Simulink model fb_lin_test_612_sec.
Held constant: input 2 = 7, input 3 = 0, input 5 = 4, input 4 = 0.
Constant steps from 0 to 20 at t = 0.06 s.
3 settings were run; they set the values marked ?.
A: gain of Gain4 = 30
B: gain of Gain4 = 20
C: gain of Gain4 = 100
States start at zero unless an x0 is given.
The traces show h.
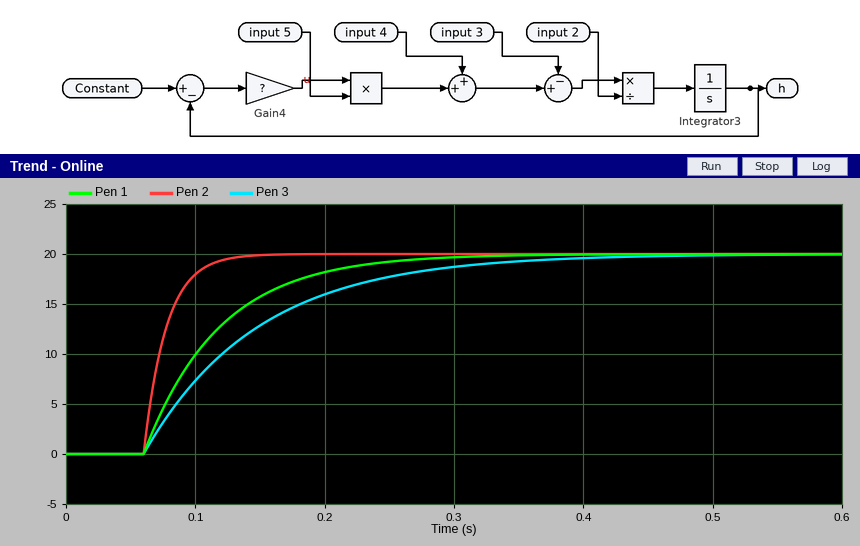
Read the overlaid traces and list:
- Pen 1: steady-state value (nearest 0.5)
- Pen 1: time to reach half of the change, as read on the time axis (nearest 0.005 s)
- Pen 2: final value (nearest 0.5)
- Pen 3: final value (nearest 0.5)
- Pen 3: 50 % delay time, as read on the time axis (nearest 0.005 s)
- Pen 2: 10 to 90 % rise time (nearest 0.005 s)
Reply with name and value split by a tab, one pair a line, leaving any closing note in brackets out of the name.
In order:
Pen 1: steady-state value	20.0
Pen 1: time to reach half of the change, as read on the time axis	0.100 s
Pen 2: final value	20.0
Pen 3: final value	20.0
Pen 3: 50 % delay time, as read on the time axis	0.120 s
Pen 2: 10 to 90 % rise time	0.040 s
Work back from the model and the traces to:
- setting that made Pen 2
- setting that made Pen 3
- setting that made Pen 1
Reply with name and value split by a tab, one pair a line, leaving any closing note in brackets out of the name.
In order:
setting that made Pen 2	C
setting that made Pen 3	B
setting that made Pen 1	A
